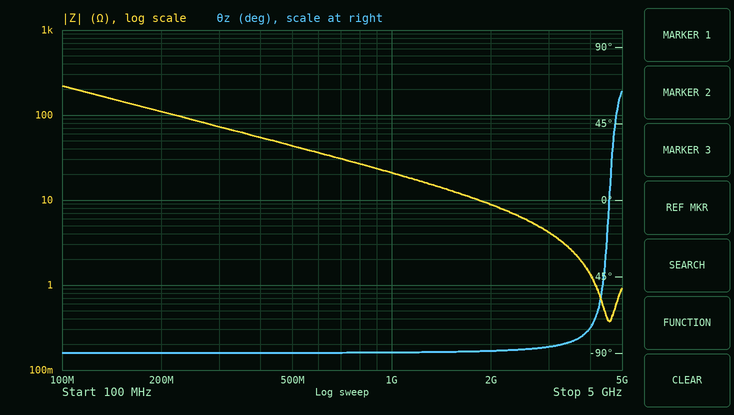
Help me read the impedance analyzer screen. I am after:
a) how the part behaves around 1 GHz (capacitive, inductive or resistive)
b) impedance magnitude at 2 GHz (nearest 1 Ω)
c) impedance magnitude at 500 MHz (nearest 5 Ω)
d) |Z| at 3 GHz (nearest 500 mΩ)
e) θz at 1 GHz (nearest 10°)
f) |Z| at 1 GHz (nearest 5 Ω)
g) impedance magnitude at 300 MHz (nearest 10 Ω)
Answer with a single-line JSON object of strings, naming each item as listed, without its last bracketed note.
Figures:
{"how the part behaves around 1 GHz": "capacitive", "impedance magnitude at 2 GHz": "9 Ω", "impedance magnitude at 500 MHz": "45 Ω", "|Z| at 3 GHz": "4.0 Ω", "θz at 1 GHz": "-90°", "|Z| at 1 GHz": "20 Ω", "impedance magnitude at 300 MHz": "70 Ω"}
